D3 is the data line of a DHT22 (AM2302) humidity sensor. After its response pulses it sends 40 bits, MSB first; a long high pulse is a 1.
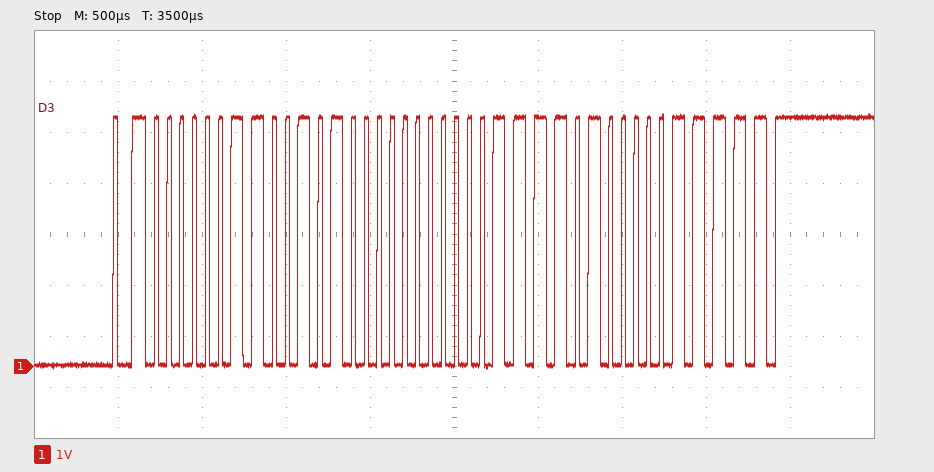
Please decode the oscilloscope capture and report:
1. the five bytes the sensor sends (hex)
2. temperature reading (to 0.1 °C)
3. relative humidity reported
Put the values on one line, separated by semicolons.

03 28 00 F4 1F; 24.4 °C; 80.8 %
